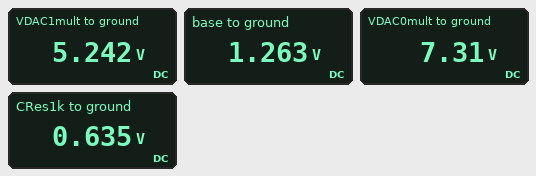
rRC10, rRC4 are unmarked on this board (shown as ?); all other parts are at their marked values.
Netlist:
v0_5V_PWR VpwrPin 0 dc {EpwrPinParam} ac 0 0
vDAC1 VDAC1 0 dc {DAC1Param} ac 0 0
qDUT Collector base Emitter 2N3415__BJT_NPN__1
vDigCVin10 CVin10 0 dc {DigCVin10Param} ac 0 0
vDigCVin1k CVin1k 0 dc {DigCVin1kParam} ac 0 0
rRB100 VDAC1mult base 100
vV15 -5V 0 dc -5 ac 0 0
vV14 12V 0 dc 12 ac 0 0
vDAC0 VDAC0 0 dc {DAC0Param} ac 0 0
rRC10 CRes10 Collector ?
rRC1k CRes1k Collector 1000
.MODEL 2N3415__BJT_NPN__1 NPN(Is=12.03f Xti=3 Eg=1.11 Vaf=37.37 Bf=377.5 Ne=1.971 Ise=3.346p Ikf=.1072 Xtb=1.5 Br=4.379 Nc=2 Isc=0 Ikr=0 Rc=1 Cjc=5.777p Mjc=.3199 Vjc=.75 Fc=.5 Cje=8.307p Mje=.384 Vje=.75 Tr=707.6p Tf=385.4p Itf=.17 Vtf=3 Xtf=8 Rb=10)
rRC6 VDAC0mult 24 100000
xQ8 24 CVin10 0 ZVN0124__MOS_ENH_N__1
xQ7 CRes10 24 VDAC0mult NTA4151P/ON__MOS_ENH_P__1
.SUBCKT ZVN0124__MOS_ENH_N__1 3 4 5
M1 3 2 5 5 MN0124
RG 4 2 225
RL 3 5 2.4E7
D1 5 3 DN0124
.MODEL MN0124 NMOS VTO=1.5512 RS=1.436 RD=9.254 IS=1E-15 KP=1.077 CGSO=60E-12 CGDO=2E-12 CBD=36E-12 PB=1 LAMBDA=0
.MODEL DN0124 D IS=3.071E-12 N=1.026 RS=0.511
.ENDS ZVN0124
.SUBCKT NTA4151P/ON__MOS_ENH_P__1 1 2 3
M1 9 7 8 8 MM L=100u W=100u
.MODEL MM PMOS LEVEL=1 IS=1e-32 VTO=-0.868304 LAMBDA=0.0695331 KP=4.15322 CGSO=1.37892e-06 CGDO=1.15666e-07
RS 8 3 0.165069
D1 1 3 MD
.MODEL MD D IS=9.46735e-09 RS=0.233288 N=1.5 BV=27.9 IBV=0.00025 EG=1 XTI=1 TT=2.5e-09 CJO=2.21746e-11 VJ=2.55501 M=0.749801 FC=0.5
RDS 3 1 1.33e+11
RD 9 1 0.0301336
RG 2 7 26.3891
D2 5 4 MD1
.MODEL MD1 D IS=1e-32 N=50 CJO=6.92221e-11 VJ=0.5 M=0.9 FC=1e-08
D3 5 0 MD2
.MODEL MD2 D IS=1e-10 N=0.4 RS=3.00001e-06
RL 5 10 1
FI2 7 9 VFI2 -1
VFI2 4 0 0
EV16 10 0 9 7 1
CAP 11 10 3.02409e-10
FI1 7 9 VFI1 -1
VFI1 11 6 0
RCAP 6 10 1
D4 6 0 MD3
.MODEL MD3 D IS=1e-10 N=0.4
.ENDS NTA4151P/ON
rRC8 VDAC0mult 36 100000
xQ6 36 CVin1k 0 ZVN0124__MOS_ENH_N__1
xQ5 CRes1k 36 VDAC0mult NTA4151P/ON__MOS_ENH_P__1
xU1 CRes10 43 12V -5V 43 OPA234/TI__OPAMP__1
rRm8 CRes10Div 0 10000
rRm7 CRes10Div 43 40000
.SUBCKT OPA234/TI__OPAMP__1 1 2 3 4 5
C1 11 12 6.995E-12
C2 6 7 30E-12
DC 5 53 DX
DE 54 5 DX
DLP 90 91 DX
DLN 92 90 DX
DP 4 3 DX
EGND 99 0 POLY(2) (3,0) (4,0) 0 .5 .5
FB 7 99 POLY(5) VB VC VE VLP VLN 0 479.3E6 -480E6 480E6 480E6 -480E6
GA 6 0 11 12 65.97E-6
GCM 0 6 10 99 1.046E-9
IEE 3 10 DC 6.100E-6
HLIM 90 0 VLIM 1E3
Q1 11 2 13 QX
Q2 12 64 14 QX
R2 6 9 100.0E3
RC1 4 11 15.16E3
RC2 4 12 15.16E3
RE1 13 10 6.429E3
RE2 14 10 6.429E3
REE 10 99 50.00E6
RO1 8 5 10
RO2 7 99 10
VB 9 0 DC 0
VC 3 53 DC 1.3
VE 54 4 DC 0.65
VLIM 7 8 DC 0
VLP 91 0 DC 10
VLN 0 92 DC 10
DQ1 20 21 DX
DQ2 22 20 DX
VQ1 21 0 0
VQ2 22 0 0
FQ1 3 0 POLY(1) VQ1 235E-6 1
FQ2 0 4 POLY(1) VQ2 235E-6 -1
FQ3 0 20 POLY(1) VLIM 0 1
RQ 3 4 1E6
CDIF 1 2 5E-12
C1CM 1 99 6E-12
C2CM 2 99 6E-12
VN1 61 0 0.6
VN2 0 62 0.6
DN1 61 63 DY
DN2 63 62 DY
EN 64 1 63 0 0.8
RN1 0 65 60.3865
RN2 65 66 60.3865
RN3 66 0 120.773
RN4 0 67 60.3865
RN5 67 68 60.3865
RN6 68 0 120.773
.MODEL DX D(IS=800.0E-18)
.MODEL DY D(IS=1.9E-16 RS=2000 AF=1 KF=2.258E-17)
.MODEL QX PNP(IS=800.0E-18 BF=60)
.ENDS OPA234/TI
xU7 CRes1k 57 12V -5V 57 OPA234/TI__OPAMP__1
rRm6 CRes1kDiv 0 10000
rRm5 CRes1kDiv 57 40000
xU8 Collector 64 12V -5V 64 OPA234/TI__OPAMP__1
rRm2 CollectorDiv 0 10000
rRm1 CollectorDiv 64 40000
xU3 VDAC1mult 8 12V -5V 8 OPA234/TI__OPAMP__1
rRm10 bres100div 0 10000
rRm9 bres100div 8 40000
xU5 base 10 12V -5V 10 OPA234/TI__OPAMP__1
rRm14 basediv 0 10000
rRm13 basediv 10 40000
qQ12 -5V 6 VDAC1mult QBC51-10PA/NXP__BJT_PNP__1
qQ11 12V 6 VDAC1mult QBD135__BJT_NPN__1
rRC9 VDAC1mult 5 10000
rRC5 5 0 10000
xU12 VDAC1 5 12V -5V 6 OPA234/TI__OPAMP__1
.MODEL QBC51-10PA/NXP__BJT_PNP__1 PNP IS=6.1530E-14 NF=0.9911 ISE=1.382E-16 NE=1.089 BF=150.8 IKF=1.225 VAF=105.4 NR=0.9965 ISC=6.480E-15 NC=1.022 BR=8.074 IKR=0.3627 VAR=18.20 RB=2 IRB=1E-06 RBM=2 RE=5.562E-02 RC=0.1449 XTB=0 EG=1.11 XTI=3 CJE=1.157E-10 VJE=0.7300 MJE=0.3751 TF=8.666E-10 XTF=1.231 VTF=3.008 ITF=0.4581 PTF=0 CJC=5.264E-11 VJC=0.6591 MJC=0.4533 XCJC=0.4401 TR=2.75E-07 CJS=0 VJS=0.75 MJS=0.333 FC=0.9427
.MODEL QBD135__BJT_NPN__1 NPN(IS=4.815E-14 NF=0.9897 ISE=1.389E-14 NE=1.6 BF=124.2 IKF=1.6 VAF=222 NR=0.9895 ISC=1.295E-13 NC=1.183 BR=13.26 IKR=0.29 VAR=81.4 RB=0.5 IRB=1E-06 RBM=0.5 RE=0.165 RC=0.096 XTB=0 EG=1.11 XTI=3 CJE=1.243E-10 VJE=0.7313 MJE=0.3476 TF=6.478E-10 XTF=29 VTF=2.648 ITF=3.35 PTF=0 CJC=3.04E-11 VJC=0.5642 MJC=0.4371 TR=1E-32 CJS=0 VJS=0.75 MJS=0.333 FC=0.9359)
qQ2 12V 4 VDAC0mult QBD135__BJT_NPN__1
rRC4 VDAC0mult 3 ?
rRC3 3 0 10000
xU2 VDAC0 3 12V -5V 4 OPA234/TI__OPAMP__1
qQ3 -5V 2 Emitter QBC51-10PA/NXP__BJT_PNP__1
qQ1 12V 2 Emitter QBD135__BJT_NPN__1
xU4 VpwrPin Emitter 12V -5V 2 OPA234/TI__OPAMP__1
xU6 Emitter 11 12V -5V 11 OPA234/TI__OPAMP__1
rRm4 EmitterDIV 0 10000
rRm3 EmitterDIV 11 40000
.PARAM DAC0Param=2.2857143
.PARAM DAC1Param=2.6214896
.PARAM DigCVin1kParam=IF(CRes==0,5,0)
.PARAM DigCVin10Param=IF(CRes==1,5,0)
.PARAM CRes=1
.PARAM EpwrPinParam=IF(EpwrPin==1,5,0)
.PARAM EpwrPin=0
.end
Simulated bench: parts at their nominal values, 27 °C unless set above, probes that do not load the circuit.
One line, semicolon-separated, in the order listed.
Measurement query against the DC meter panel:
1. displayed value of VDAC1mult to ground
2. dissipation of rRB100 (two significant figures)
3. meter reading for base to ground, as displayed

5.242 V; 160 mW; 1.263 V
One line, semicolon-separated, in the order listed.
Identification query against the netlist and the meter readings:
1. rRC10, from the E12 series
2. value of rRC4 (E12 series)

12 Ω; 22 kΩ
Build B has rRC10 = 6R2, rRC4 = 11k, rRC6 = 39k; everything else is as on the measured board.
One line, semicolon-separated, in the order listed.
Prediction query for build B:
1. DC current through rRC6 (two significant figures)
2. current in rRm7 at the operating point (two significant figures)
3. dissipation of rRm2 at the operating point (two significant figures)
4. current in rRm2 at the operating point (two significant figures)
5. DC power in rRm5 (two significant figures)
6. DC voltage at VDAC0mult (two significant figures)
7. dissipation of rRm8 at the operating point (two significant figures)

120 µA; 93 µA; 2.1 µW; 15 µA; 8.5 µW; 4.8 V; 86 µW
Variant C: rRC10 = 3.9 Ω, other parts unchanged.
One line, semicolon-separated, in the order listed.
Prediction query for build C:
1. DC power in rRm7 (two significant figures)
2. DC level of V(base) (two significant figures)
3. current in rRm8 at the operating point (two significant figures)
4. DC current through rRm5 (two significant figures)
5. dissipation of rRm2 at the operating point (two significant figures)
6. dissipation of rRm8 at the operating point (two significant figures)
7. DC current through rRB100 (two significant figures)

430 µW; 1.9 V; 100 µA; 35 µA; 12 µW; 110 µW; 33 mA
